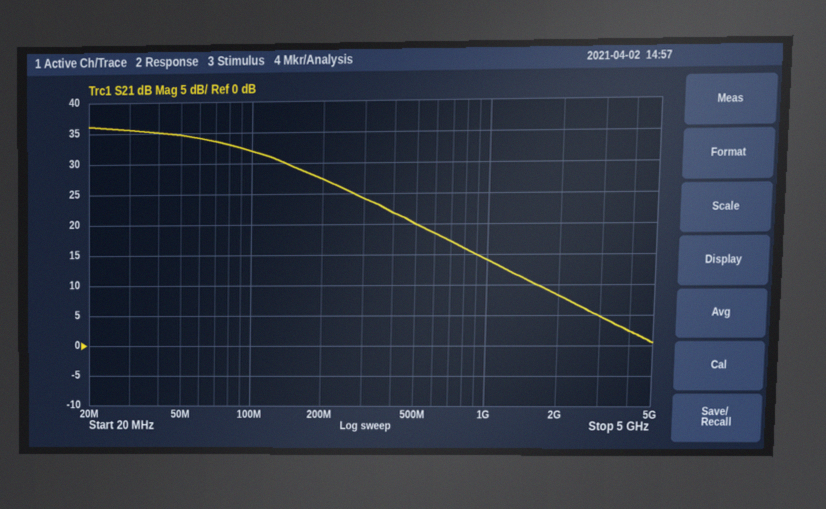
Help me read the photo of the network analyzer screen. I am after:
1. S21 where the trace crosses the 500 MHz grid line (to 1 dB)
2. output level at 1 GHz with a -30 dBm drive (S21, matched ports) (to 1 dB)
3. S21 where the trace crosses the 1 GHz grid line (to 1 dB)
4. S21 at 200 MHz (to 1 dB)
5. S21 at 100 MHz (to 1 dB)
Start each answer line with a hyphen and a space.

- 20 dB
- -16 dBm
- 14 dB
- 27 dB
- 32 dB
